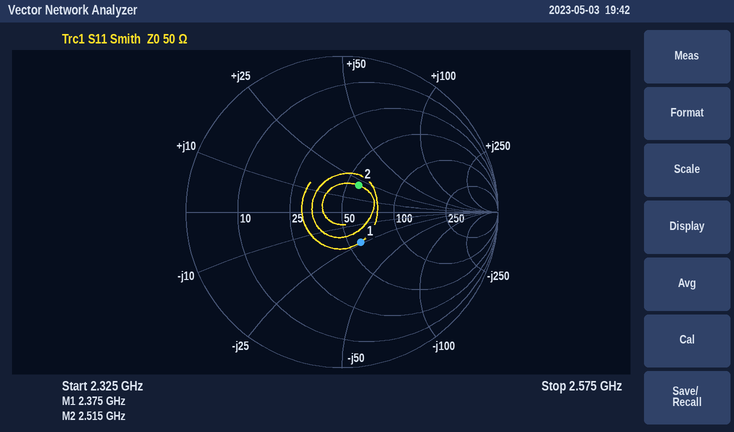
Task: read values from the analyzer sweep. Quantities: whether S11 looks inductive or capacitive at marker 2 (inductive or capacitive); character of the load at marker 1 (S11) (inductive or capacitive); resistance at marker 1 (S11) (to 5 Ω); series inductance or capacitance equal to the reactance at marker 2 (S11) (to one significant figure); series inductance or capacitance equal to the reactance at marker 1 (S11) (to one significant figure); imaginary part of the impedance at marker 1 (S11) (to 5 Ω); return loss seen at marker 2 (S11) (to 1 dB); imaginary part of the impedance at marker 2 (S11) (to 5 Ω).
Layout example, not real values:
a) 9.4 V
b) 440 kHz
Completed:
a) inductive
b) capacitive
c) 60 Ω
d) 1 nH
e) 3 pF
f) -25 Ω
g) 14 dB
h) +20 Ω
